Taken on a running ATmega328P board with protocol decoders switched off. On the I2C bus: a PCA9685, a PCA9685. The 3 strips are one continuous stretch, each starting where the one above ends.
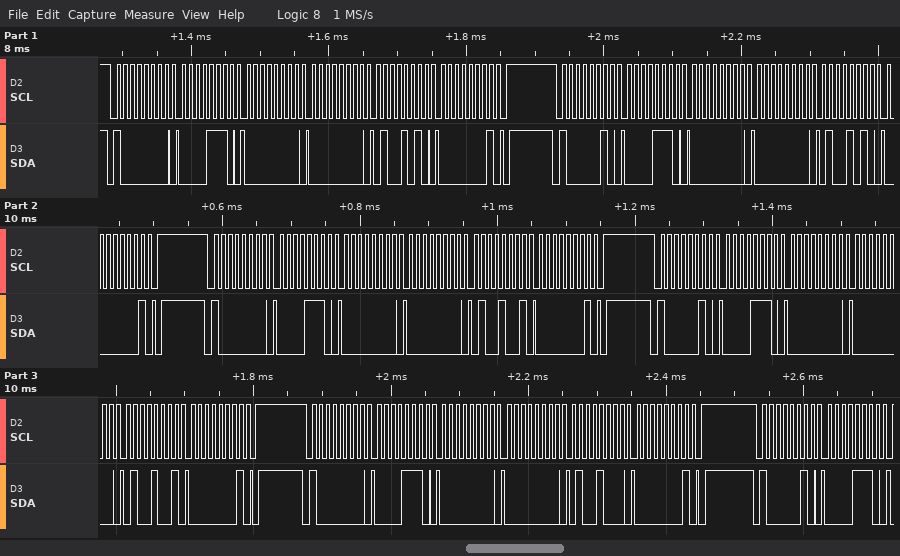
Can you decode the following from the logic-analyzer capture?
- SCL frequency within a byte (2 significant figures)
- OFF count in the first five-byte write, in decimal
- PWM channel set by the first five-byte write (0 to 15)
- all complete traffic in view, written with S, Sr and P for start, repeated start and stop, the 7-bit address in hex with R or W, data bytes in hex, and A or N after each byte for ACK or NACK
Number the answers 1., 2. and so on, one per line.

1. 100 kHz
2. 330
3. 2
4. S 40W A 0E A 00 A 00 A 4A A 01 A P S 41W A 0E A 00 A 00 A 4A A 01 A P S 40W A 0E A 00 A 00 A 49 A 01 A P S 41W A 0E A 00 A 00 A 49 A 01 A P S 40W A 0E A 00 A 00 A 48 A 01 A P S 41W A 0E A
